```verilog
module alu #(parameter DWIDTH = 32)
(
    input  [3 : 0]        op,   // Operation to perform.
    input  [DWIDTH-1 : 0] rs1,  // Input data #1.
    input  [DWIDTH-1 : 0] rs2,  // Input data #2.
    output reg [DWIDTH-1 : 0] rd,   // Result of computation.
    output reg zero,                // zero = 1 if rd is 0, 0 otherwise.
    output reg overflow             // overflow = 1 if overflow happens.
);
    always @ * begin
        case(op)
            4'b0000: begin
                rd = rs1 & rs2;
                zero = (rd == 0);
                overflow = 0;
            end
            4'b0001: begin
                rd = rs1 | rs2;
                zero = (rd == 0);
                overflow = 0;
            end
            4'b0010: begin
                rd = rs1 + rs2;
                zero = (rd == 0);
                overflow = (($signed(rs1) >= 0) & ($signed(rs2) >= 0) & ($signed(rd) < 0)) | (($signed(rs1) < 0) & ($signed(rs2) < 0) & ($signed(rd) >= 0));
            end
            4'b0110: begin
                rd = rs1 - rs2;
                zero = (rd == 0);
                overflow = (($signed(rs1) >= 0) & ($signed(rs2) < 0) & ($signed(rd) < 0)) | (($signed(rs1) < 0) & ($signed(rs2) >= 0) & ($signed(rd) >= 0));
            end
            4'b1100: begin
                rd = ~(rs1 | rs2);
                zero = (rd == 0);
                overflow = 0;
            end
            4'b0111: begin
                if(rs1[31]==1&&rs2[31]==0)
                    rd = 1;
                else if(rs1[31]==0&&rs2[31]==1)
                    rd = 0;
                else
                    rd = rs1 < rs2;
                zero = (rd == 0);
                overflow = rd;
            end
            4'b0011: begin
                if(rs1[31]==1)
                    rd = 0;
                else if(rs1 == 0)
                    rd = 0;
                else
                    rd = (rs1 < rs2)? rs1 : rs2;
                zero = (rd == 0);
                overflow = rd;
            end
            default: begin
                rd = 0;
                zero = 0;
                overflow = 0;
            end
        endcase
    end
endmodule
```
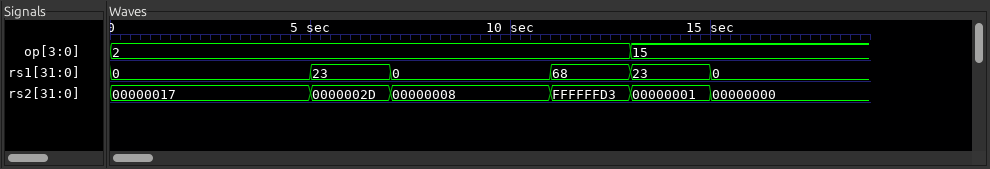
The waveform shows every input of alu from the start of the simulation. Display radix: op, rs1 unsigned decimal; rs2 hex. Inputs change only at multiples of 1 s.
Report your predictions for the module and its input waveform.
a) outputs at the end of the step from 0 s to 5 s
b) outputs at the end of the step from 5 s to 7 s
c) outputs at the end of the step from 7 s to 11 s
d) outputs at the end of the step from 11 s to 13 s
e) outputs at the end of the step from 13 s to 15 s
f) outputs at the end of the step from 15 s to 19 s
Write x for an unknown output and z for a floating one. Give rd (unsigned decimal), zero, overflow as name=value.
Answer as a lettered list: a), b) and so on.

a) rd=23, zero=0, overflow=0
b) rd=68, zero=0, overflow=0
c) rd=8, zero=0, overflow=0
d) rd=23, zero=0, overflow=0
e) rd=0, zero=0, overflow=0
f) rd=0, zero=0, overflow=0
